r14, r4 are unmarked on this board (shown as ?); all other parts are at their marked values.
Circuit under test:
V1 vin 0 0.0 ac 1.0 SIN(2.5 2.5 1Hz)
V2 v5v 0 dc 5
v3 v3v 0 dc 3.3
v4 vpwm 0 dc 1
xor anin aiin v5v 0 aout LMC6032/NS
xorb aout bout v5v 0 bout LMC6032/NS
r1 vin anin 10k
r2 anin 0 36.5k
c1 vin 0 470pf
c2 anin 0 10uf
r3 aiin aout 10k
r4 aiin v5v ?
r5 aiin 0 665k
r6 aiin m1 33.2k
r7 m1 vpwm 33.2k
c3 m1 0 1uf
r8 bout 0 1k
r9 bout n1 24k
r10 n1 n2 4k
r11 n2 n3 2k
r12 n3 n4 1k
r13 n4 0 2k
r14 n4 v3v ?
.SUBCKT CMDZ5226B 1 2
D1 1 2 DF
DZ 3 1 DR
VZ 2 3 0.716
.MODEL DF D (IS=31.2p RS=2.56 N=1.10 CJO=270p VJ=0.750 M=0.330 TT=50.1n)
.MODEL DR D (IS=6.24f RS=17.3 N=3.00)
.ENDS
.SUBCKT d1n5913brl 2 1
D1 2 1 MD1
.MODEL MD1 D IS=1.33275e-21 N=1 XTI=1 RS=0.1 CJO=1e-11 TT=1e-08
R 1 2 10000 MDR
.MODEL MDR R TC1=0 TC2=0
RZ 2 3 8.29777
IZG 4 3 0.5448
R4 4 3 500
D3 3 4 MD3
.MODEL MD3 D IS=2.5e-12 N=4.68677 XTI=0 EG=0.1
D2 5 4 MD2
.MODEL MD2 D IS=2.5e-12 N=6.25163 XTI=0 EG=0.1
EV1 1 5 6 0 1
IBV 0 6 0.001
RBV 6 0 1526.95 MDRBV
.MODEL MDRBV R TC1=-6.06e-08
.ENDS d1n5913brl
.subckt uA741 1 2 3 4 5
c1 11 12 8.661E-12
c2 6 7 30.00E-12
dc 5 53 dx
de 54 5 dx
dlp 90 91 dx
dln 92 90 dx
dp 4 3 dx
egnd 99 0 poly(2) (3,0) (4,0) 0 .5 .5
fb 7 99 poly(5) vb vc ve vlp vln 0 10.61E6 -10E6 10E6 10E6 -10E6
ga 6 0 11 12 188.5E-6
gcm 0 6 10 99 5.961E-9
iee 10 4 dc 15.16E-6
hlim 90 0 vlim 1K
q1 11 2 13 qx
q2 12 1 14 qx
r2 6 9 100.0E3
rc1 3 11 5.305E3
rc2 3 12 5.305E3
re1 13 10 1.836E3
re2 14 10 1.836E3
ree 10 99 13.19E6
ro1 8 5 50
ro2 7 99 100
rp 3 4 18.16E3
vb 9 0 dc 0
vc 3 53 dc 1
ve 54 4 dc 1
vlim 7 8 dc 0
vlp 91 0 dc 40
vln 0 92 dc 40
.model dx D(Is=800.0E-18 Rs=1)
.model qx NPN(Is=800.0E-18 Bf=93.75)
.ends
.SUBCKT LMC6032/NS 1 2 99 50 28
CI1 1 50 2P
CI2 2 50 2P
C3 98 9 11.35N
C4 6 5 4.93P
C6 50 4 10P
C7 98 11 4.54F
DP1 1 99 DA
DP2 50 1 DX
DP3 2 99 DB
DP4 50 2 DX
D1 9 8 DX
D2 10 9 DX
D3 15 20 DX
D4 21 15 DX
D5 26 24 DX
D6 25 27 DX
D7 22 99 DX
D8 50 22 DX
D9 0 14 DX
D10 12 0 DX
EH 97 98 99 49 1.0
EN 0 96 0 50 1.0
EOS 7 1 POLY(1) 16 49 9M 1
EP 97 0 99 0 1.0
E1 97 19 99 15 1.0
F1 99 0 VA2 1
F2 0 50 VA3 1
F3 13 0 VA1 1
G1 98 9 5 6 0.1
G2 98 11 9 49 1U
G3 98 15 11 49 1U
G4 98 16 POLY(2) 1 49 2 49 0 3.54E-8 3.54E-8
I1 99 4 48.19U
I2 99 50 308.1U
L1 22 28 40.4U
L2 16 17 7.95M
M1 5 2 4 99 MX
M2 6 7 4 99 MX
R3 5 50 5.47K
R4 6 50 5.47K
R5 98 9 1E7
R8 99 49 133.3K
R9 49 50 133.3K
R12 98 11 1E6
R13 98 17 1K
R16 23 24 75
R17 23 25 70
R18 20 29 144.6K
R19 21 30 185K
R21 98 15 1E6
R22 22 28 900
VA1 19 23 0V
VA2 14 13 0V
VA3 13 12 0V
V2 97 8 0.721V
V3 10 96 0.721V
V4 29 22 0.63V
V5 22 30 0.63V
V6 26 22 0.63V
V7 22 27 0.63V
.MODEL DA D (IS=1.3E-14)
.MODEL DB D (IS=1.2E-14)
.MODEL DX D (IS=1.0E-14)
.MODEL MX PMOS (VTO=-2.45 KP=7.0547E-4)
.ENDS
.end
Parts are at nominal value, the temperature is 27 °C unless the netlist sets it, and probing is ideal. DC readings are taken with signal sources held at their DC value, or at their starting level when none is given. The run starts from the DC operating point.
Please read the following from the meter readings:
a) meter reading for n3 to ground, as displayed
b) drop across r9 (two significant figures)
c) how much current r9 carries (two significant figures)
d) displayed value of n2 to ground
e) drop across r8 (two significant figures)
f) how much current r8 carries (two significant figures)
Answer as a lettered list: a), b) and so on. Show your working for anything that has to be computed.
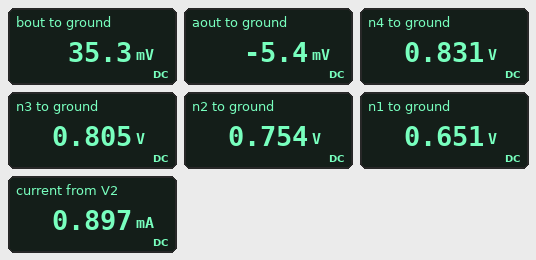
a) 0.805 V
b) 651 mV - 35.3 mV = 620 mV
c) (651 mV - 35.3 mV) / 24 kΩ = 26 µA
d) 0.754 V
e) 35.3 mV = 35 mV
f) (35.3 mV) / 1 kΩ = 35 µA
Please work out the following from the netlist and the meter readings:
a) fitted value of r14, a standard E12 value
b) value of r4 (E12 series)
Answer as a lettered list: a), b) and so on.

a) 5.6 kΩ
b) 27 kΩ
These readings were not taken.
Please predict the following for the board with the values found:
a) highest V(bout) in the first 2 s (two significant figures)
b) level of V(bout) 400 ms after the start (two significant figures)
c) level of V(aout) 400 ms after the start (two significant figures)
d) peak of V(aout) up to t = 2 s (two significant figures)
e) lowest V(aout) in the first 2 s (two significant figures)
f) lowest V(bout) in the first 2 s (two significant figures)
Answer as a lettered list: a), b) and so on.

a) 2.8 V
b) 2.8 V
c) 2.8 V
d) 2.8 V
e) -5.4 mV
f) 35 mV
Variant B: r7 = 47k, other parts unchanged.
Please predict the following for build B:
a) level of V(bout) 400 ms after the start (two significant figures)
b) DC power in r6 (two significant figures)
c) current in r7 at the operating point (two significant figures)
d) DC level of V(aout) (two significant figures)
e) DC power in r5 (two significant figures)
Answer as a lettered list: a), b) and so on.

a) 2.7 V
b) 480 nW
c) 3.8 µA
d) -5.3 mV
e) 2.6 µW
